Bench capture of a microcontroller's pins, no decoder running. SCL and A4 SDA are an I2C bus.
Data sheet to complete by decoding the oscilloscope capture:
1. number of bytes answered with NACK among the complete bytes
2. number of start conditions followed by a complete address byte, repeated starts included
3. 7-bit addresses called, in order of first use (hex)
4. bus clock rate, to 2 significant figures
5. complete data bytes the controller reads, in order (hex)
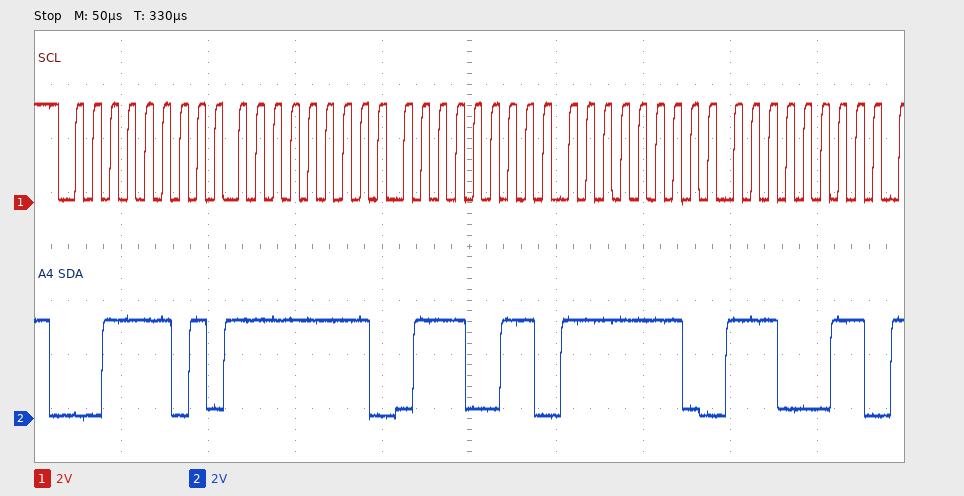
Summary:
0
1
0x1E
100 kHz
FF 73 FE E3
